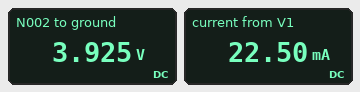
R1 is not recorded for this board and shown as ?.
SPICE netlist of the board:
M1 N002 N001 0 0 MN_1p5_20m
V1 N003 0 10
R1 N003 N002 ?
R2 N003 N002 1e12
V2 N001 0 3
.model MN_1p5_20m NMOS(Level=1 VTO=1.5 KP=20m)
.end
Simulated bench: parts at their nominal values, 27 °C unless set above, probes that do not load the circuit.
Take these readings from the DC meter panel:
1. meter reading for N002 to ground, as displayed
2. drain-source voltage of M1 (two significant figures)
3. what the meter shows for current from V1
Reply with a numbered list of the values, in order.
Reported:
1. 3.925 V
2. 3.9 V
3. 22.50 mA
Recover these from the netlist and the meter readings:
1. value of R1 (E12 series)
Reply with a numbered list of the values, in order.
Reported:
1. 270 Ω
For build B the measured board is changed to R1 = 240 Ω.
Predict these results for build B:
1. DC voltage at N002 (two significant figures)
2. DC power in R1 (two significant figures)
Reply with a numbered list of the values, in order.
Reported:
1. 4.6 V
2. 120 mW
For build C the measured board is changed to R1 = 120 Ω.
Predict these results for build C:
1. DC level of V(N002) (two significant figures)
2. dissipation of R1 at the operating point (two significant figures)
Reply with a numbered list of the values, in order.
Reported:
1. 7.3 V
2. 61 mW
